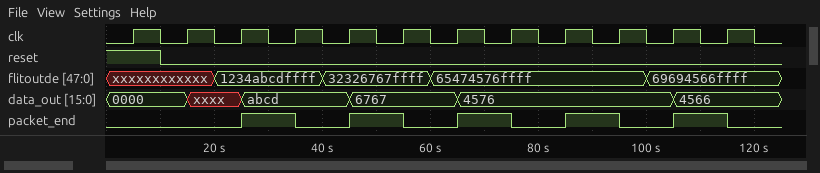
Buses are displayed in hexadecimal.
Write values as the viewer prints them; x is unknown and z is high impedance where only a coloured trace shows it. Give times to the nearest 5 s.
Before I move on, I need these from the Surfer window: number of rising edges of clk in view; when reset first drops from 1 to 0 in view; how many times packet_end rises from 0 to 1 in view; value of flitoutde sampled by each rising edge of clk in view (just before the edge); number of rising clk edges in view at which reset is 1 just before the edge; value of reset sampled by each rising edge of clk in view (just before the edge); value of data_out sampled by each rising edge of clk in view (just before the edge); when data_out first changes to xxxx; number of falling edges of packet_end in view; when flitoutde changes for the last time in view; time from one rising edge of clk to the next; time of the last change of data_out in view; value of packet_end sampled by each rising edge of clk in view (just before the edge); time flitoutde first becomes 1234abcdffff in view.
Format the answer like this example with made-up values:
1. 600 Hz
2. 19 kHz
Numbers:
1. 12
2. 10 s
3. 5
4. xxxxxxxxxxxx, xxxxxxxxxxxx, 1234abcdffff, 1234abcdffff, 32326767ffff, 32326767ffff, 65474576ffff, 65474576ffff, 65474576ffff, 65474576ffff, 69694566ffff, 69694566ffff
5. 1
6. 1 0 0 0 0 0 0 0 0 0 0 0
7. 0000, 0000, xxxx, abcd, abcd, 6767, 6767, 4576, 4576, 4576, 4576, 4566
8. 15 s
9. 5
10. 100 s
11. 10 s
12. 105 s
13. 0 0 0 1 0 1 0 1 0 1 0 1
14. 20 s
